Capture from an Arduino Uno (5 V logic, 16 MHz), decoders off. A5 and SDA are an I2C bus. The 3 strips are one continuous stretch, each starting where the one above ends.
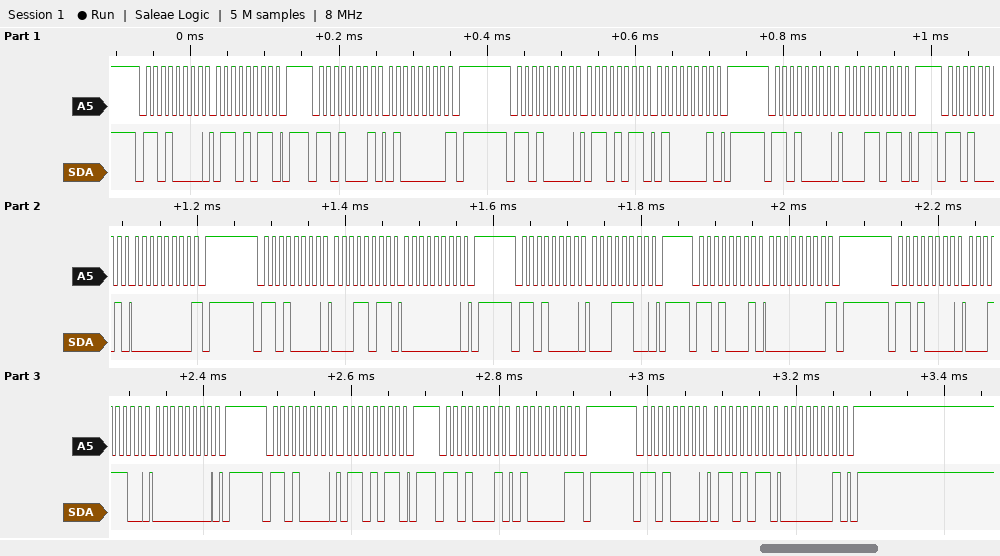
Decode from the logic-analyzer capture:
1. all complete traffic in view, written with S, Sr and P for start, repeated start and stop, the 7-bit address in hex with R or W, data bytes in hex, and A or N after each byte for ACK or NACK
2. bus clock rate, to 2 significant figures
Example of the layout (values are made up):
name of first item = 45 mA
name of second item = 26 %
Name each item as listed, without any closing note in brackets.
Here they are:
all complete traffic in view, written with S, Sr and P for start, repeated start and stop, the 7-bit address in hex with R or W, data bytes in hex, and A or N after each byte for ACK or NACK = S 68W A 6B A P S 68R A 40 N P S 68W A 6B A 41 A P S 68W A 1B A P S 68R A 00 N P S 68W A 1B A 00 A P S 68W A 1C A P S 68R A 00 N P S 68W A 1C A 00 A P S 68W A 6B A P S 68R A 41 N P S 68W A 6B A 01 A P
bus clock rate, to 2 significant figures = 100 kHz
